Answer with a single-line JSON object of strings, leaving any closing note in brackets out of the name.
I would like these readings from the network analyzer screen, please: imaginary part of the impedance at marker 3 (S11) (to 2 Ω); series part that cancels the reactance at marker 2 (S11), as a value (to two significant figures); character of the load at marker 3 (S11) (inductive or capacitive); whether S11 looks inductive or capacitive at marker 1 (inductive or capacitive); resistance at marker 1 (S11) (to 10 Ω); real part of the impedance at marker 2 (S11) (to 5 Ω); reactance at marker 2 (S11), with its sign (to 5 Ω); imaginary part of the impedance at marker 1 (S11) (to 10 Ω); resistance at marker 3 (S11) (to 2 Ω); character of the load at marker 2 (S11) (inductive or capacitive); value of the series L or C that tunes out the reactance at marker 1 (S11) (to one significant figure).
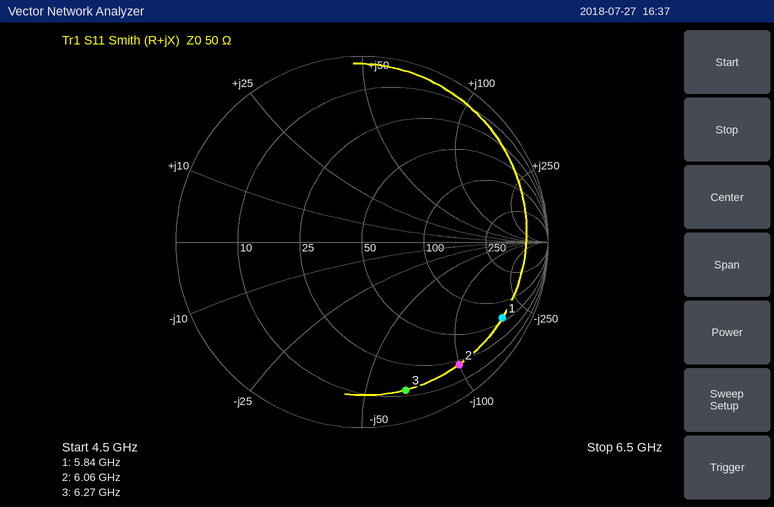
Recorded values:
{"imaginary part of the impedance at marker 3 (S11)": "-66 Ω", "series part that cancels the reactance at marker 2 (S11), as a value": "2.6 nH", "character of the load at marker 3 (S11)": "capacitive", "whether S11 looks inductive or capacitive at marker 1": "capacitive", "resistance at marker 1 (S11)": "60 Ω", "real part of the impedance at marker 2 (S11)": "20 Ω", "reactance at marker 2 (S11), with its sign": "-100 Ω", "imaginary part of the impedance at marker 1 (S11)": "-180 Ω", "resistance at marker 3 (S11)": "12 Ω", "character of the load at marker 2 (S11)": "capacitive", "value of the series L or C that tunes out the reactance at marker 1 (S11)": "5 nH"}
